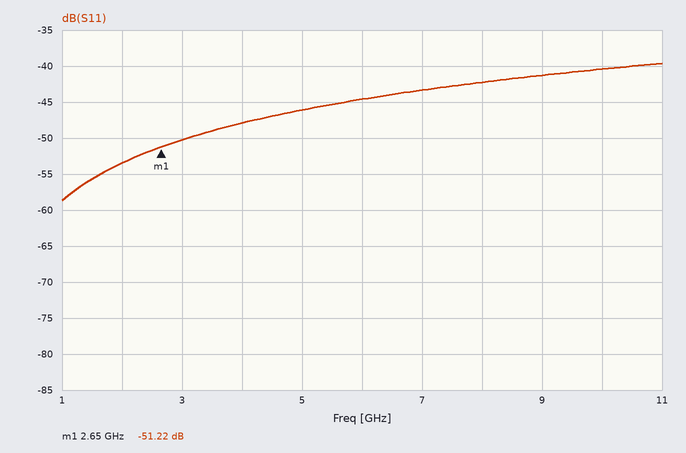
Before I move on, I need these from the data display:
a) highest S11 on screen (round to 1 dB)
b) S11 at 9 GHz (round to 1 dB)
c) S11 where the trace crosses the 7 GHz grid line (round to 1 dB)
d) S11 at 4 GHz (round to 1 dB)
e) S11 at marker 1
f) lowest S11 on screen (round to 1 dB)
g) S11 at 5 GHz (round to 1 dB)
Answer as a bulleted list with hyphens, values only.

- -40 dB
- -41 dB
- -43 dB
- -48 dB
- -51.22 dB
- -59 dB
- -46 dB
